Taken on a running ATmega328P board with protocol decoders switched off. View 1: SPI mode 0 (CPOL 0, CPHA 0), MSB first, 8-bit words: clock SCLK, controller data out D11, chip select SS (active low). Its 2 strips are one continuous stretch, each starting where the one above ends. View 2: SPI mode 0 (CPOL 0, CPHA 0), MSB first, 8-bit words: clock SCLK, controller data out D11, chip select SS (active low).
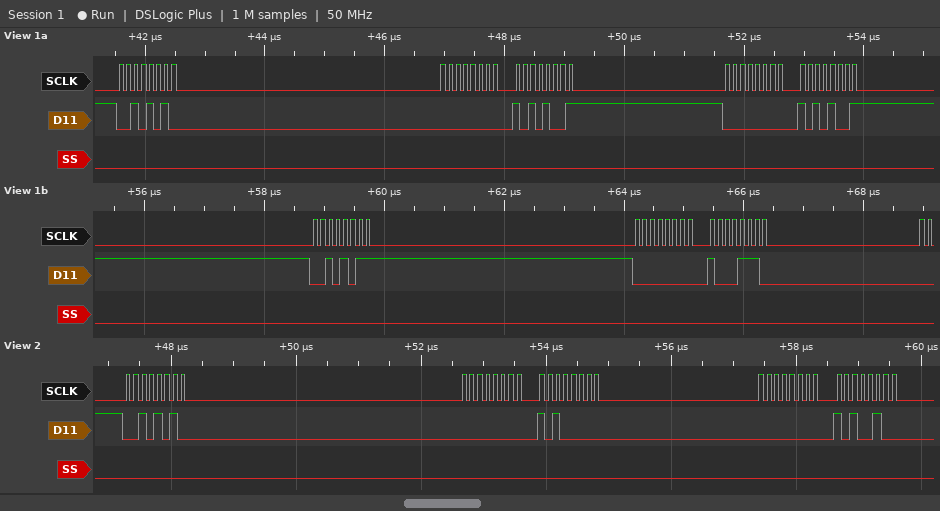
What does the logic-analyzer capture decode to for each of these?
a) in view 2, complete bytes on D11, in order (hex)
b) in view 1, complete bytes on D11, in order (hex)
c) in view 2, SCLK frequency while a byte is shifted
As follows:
2A 00 A0 00 A4
2A 00 A9 00 A9 2B 00 8E
8 MHz
